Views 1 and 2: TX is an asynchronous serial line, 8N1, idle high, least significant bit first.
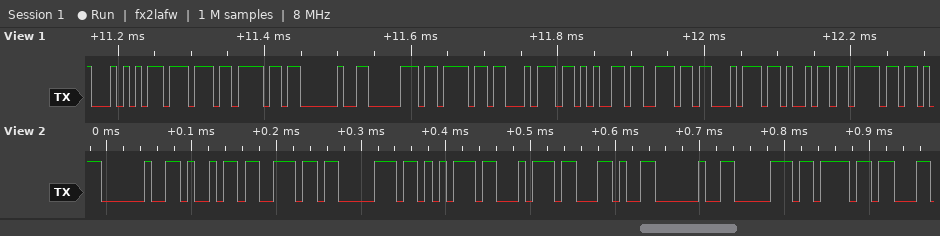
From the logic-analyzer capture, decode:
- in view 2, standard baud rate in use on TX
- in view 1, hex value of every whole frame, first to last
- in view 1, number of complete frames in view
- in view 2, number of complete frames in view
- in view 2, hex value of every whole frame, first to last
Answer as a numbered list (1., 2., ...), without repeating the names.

1. 115200 baud
2. 54 77 6F 20 70 6F 74 65 6E 74 69 6F
3. 12
4. 10
5. 20 69 6E 70 75 74 2C 20 70 6F
